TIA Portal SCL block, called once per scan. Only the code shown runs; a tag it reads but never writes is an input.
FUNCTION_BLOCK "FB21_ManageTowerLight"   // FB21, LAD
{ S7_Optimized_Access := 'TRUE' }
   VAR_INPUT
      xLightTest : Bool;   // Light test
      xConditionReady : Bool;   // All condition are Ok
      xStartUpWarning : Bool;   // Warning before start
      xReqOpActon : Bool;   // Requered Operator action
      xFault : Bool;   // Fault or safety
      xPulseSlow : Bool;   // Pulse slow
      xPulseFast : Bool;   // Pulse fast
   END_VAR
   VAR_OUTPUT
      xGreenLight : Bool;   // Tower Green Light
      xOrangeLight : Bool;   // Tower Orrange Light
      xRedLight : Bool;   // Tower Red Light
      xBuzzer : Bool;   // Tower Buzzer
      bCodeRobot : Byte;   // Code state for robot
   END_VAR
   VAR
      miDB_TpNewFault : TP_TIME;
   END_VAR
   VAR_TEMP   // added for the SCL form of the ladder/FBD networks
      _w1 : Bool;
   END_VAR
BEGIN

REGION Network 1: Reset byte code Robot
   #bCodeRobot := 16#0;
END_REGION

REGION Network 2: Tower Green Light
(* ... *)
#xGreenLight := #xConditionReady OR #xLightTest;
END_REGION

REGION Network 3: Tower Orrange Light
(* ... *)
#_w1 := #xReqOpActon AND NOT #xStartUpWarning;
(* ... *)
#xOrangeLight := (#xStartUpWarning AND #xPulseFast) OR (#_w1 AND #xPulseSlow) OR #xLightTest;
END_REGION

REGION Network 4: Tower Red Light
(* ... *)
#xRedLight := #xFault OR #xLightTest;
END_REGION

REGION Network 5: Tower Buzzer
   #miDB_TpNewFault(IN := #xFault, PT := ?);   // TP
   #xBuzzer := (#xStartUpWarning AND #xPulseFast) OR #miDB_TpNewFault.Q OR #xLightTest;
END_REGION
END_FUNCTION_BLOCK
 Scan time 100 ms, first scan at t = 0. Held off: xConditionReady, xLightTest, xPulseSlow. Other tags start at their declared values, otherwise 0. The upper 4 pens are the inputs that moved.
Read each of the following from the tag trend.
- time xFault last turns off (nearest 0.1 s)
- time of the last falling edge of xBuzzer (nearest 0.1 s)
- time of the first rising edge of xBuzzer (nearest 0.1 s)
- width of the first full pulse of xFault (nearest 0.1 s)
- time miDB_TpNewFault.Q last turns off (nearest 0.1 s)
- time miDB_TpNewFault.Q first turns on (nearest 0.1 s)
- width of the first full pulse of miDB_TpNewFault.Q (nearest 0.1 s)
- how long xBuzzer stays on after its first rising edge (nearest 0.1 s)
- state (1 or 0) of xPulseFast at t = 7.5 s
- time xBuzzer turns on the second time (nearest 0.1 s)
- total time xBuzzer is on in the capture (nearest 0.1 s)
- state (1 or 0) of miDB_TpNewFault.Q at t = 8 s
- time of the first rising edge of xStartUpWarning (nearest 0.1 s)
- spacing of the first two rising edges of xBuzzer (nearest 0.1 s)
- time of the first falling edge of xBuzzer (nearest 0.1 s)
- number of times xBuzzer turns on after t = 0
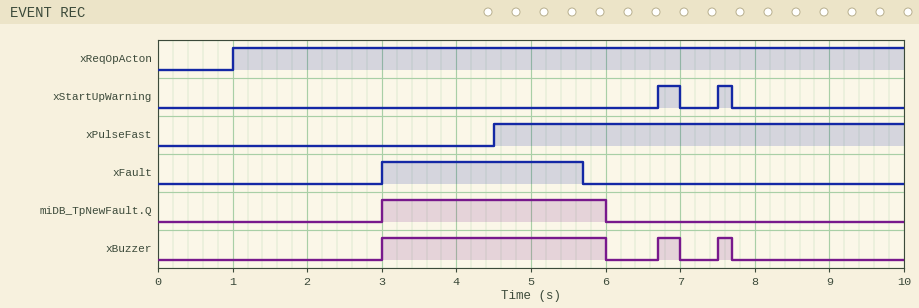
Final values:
5.7 s
7.7 s
3.0 s
2.7 s
6.0 s
3.0 s
3.0 s
3.0 s
1
6.7 s
3.5 s
0
6.7 s
3.7 s
6.0 s
3
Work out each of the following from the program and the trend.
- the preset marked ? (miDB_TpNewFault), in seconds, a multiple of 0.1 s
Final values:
3.0 s
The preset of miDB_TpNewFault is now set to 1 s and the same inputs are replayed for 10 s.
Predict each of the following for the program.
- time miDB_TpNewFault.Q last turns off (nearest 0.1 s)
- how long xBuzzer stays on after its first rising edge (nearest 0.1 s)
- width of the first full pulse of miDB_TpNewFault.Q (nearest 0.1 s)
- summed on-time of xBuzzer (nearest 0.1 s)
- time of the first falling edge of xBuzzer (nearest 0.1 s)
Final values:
4.0 s
1.0 s
1.0 s
1.5 s
4.0 s
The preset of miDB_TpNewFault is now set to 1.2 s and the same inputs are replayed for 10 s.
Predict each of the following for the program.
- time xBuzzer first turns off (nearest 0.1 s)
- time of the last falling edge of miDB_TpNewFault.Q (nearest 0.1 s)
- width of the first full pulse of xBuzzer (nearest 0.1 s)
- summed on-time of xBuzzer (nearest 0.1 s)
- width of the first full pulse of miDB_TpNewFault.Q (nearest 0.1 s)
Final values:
4.2 s
4.2 s
1.2 s
1.7 s
1.2 s
